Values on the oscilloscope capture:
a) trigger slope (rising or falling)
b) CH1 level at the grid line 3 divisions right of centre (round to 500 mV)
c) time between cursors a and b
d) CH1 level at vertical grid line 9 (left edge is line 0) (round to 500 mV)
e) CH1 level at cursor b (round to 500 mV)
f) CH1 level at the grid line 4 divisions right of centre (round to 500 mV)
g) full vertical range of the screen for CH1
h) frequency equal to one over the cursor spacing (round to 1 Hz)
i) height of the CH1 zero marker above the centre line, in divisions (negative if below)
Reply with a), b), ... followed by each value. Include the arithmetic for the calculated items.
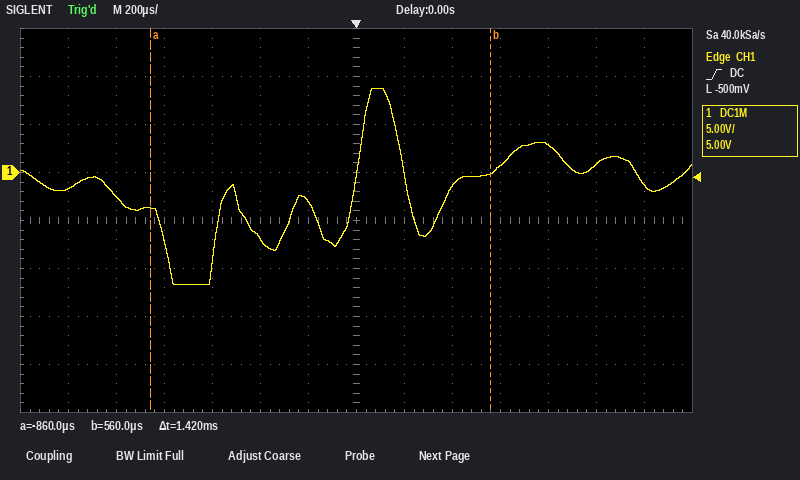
a) rising
b) 500 mV
c) 1.42 ms
d) -1.5 V
e) 0.0 V
f) 3.0 V
g) 40 V
h) 1 / 1.42 ms ≈ 704 Hz
i) +1.0 div
